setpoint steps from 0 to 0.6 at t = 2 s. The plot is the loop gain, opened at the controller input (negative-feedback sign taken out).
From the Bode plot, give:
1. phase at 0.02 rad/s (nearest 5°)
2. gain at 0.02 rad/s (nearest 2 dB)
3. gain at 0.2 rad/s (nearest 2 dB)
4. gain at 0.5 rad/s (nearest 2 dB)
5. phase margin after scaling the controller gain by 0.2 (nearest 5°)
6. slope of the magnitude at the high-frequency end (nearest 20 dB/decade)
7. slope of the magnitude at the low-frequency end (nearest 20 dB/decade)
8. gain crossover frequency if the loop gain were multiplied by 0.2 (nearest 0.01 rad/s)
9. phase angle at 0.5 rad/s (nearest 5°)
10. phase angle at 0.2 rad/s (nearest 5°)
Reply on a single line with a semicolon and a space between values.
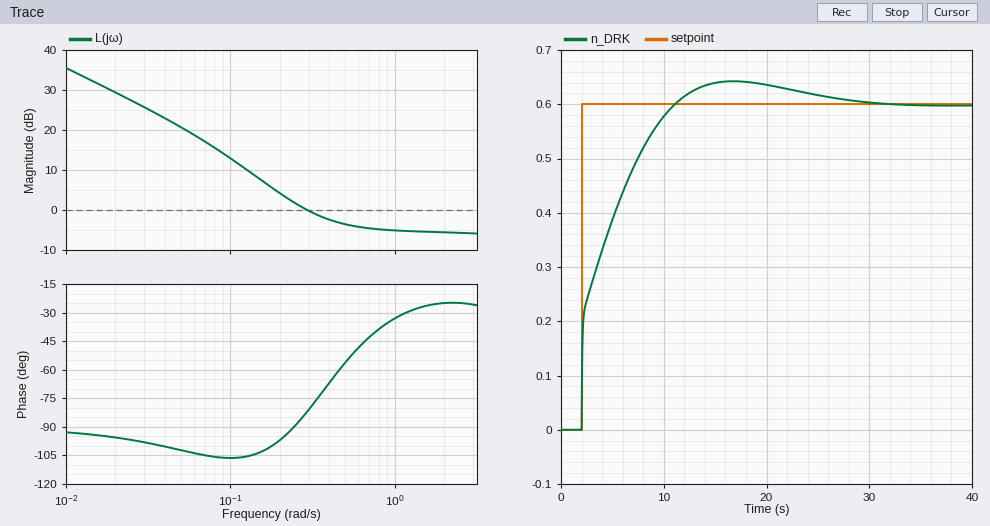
-95°; 30 dB; 4 dB; -4 dB; 75°; 0 dB/decade; -20 dB/decade; 0.09 rad/s; -55°; -95°
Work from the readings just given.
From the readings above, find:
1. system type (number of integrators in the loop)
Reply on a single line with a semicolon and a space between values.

1
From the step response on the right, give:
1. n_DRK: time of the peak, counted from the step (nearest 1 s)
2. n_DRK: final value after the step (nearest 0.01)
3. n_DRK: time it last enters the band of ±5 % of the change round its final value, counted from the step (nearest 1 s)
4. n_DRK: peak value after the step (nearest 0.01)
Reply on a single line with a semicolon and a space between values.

15 s; 0.60; 20 s; 0.64
